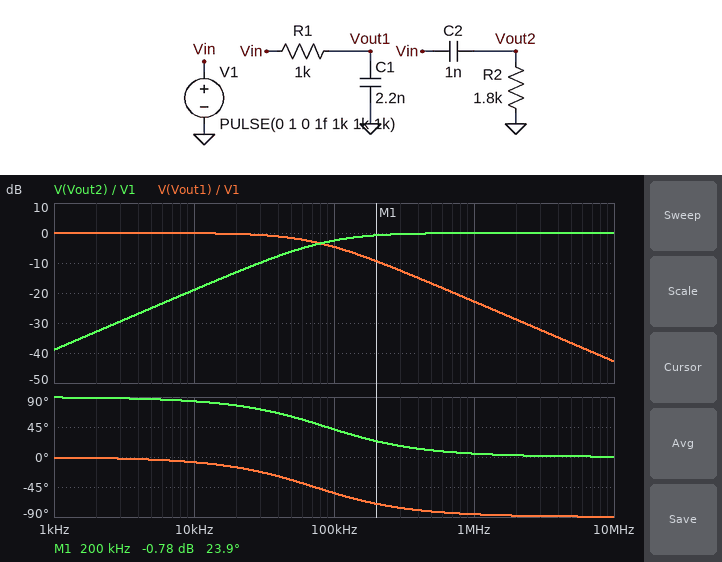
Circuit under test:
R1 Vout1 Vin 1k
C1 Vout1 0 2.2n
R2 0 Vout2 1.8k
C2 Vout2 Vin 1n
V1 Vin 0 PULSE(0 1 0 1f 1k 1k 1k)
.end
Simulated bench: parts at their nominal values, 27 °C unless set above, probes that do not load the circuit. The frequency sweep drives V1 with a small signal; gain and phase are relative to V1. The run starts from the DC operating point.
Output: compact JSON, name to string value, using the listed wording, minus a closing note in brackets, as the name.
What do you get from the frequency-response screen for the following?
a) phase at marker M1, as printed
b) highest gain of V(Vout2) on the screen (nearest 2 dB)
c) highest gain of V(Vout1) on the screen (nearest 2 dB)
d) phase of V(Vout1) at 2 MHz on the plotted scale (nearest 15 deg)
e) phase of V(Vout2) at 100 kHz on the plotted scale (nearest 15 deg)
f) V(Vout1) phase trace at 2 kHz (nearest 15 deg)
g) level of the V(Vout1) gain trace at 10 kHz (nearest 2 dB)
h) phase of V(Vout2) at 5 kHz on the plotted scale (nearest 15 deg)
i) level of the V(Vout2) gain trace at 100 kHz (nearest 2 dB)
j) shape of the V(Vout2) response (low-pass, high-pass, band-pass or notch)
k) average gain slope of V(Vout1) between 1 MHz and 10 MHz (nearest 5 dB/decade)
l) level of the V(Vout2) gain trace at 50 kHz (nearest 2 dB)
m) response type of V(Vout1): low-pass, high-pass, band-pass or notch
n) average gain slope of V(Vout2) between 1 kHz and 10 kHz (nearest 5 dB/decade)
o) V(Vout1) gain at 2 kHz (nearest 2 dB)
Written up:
{"phase at marker M1, as printed": "23.9 deg", "highest gain of V(Vout2) on the screen": "0 dB", "highest gain of V(Vout1) on the screen": "0 dB", "phase of V(Vout1) at 2 MHz on the plotted scale": "-90 deg", "phase of V(Vout2) at 100 kHz on the plotted scale": "45 deg", "V(Vout1) phase trace at 2 kHz": "0 deg", "level of the V(Vout1) gain trace at 10 kHz": "0 dB", "phase of V(Vout2) at 5 kHz on the plotted scale": "90 deg", "level of the V(Vout2) gain trace at 100 kHz": "-2 dB", "shape of the V(Vout2) response": "high-pass", "average gain slope of V(Vout1) between 1 MHz and 10 MHz": "-20 dB/decade", "level of the V(Vout2) gain trace at 50 kHz": "-6 dB", "response type of V(Vout1): low-pass, high-pass, band-pass or notch": "low-pass", "average gain slope of V(Vout2) between 1 kHz and 10 kHz": "20 dB/decade", "V(Vout1) gain at 2 kHz": "0 dB"}
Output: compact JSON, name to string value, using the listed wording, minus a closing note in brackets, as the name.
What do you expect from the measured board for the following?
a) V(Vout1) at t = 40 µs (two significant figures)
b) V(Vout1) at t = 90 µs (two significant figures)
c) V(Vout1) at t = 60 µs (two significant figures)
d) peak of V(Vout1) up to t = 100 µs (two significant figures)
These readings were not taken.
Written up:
{"V(Vout1) at t = 40 µs": "1.0 V", "V(Vout1) at t = 90 µs": "1.0 V", "V(Vout1) at t = 60 µs": "1.0 V", "peak of V(Vout1) up to t = 100 µs": "1.0 V"}
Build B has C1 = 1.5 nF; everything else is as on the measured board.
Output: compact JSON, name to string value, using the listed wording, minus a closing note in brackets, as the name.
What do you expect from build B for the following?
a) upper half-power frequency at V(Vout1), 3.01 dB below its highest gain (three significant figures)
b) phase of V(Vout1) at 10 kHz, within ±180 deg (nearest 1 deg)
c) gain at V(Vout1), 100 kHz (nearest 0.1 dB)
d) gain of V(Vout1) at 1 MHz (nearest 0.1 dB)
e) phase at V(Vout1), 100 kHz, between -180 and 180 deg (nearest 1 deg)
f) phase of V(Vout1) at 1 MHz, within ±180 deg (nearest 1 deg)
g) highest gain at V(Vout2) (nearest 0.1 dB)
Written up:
{"upper half-power frequency at V(Vout1), 3.01 dB below its highest gain": "106 kHz", "phase of V(Vout1) at 10 kHz, within ±180 deg": "-5 deg", "gain at V(Vout1), 100 kHz": "-2.8 dB", "gain of V(Vout1) at 1 MHz": "-19.5 dB", "phase at V(Vout1), 100 kHz, between -180 and 180 deg": "-43 deg", "phase of V(Vout1) at 1 MHz, within ±180 deg": "-84 deg", "highest gain at V(Vout2)": "0 dB"}
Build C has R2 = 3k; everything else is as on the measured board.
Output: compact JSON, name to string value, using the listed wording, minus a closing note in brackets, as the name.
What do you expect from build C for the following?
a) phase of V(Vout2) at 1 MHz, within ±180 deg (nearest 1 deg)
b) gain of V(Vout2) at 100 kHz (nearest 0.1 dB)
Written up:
{"phase of V(Vout2) at 1 MHz, within ±180 deg": "3 deg", "gain of V(Vout2) at 100 kHz": "-1.1 dB"}
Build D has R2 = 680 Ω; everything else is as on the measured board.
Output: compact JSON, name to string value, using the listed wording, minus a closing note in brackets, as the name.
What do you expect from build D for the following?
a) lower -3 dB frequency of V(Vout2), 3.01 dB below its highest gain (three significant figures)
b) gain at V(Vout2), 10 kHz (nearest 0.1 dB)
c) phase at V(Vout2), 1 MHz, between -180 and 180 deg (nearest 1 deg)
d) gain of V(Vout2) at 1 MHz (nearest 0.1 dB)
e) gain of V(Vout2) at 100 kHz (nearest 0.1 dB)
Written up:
{"lower -3 dB frequency of V(Vout2), 3.01 dB below its highest gain": "234 kHz", "gain at V(Vout2), 10 kHz": "-27.4 dB", "phase at V(Vout2), 1 MHz, between -180 and 180 deg": "13 deg", "gain of V(Vout2) at 1 MHz": "-0.2 dB", "gain of V(Vout2) at 100 kHz": "-8.1 dB"}
